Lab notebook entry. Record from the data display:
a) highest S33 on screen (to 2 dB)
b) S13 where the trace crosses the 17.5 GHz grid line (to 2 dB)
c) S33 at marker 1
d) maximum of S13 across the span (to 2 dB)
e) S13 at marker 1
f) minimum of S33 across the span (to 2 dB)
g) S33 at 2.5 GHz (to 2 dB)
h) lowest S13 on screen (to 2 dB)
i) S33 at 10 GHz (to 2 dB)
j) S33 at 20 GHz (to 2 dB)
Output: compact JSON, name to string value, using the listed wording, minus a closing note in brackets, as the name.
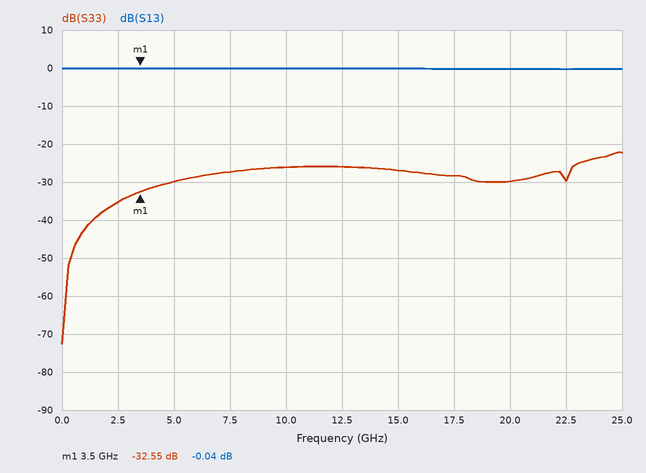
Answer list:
{"highest S33 on screen": "-22 dB", "S13 where the trace crosses the 17.5 GHz grid line": "0 dB", "S33 at marker 1": "-32.55 dB", "maximum of S13 across the span": "0 dB", "S13 at marker 1": "-0.04 dB", "minimum of S33 across the span": "-72 dB", "S33 at 2.5 GHz": "-36 dB", "lowest S13 on screen": "0 dB", "S33 at 10 GHz": "-26 dB", "S33 at 20 GHz": "-30 dB"}
